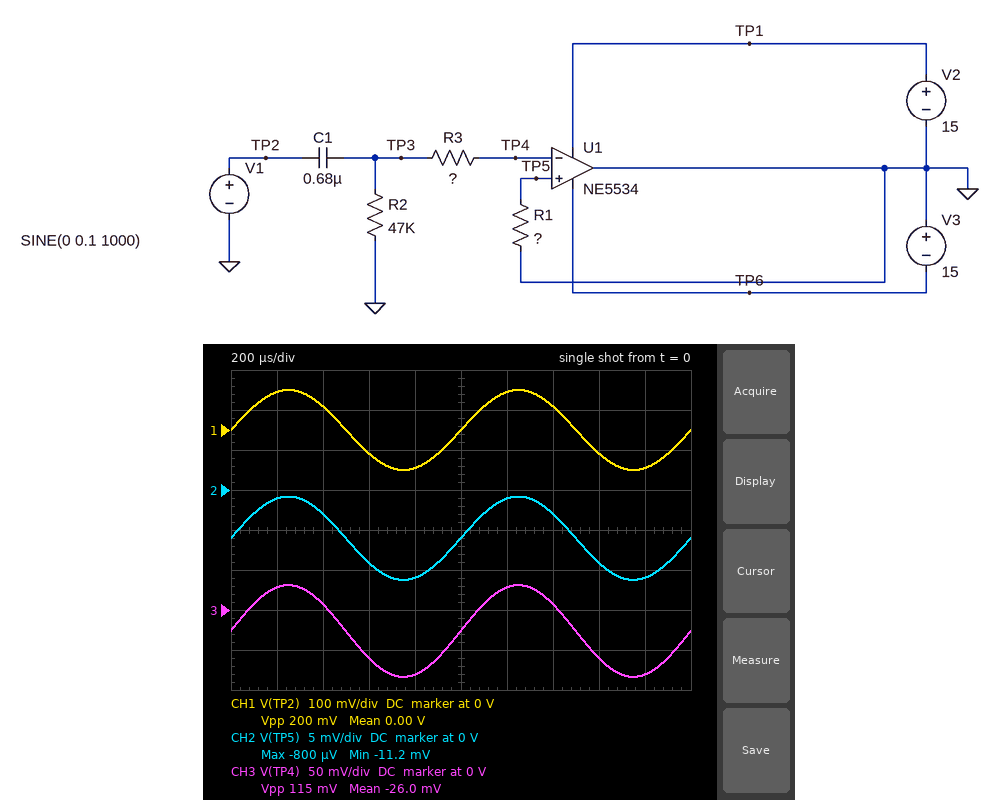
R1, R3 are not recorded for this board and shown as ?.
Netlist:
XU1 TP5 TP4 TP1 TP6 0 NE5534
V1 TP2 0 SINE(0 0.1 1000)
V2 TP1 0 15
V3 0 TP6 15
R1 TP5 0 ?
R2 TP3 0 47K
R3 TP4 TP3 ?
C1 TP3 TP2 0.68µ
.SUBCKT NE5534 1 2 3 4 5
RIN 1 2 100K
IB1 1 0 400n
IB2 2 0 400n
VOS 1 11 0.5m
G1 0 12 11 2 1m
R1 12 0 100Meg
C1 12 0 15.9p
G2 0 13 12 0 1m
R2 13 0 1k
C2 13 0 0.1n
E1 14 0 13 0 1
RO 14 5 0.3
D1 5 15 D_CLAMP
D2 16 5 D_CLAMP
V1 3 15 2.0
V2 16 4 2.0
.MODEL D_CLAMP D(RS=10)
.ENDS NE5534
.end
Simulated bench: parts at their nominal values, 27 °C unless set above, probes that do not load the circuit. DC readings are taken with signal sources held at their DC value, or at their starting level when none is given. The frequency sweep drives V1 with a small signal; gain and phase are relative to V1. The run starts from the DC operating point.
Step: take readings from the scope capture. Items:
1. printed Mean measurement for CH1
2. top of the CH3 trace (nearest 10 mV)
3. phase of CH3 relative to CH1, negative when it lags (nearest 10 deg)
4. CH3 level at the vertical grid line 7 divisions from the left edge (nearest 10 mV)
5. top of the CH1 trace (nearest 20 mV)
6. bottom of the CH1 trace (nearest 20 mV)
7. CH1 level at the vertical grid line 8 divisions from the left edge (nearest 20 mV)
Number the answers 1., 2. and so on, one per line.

1. 0.00 V
2. 30 mV
3. 0 deg
4. 10 mV
5. 100 mV
6. -100 mV
7. -60 mV
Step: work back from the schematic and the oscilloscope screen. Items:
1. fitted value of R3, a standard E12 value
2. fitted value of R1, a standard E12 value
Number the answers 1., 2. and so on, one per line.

1. 82 kΩ
2. 10 kΩ
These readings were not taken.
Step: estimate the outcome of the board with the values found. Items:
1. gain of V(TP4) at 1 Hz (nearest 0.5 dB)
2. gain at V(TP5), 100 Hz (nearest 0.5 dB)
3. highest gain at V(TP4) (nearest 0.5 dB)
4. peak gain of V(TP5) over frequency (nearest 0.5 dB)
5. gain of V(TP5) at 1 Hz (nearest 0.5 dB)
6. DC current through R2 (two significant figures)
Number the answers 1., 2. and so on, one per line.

1. -21.0 dB
2. -25.5 dB
3. -5.0 dB
4. -25.5 dB
5. -41.5 dB
6. 200 nA
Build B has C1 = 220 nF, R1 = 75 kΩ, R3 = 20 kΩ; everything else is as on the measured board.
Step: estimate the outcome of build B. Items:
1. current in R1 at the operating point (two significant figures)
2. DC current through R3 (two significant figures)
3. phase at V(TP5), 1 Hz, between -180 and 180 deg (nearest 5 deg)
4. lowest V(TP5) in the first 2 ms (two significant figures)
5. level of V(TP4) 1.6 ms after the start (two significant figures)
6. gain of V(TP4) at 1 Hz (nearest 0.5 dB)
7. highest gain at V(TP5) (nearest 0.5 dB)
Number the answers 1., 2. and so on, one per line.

1. 390 nA
2. 410 nA
3. 85 deg
4. -68 mV
5. -83 mV
6. -26.5 dB
7. -8.5 dB
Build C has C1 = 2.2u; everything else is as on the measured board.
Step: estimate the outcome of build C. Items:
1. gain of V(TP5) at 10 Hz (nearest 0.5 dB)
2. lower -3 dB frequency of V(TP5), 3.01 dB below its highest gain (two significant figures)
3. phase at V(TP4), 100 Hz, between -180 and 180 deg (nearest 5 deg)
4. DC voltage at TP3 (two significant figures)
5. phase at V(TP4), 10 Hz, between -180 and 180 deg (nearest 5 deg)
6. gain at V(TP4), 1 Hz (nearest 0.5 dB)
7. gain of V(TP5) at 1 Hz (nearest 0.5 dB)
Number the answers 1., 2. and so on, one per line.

1. -26.0 dB
2. 1.9 Hz
3. 0 deg
4. -9.4 mV
5. 10 deg
6. -11.5 dB
7. -32.5 dB
